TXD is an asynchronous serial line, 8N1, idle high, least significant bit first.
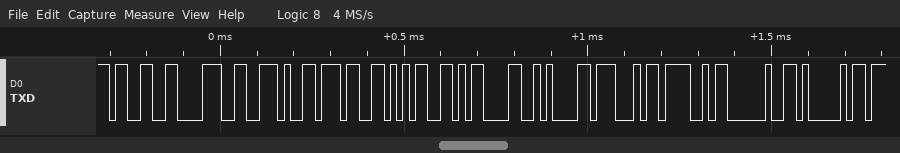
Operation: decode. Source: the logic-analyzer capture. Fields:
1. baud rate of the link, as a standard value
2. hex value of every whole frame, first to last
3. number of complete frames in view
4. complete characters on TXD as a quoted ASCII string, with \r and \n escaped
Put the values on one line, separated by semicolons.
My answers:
57600 baud; 33 38 2E 37 35 0D 0A 47 4F 20 41; 11; "38.75\r\nGO A"
